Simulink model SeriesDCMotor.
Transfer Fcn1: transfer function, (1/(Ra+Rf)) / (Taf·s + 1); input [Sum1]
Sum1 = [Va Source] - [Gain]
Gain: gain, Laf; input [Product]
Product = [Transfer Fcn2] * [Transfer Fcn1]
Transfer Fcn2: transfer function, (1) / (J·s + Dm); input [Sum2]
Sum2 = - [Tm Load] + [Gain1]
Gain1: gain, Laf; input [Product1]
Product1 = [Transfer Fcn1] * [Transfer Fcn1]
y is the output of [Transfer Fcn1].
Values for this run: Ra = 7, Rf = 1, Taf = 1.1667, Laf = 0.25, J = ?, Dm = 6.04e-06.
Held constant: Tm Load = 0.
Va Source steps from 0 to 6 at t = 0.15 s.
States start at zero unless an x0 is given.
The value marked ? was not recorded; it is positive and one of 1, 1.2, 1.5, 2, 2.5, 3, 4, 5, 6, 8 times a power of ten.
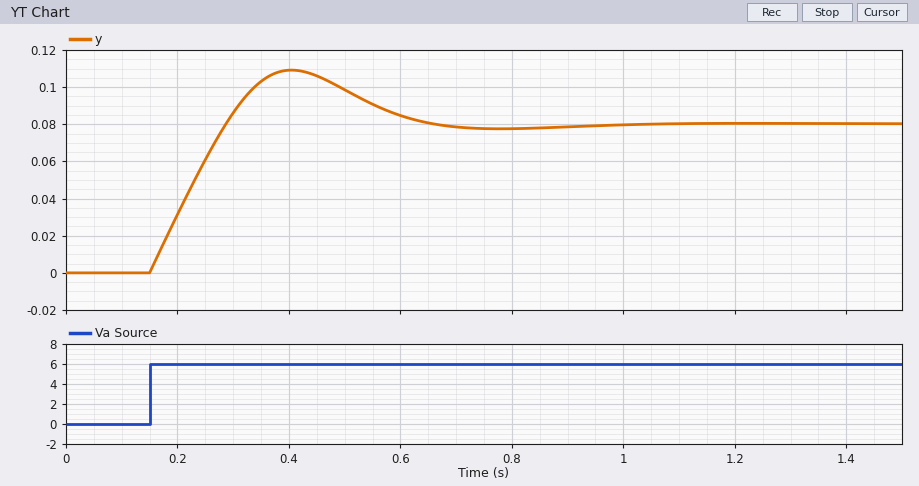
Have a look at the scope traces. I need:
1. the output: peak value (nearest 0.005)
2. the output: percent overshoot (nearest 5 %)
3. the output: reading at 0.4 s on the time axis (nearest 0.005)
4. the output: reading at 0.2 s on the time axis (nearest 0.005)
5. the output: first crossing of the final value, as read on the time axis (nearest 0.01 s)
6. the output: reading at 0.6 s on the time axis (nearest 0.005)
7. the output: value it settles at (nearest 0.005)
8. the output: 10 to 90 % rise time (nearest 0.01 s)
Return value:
0.110
35 %
0.110
0.030
0.29 s
0.085
0.080
0.11 s
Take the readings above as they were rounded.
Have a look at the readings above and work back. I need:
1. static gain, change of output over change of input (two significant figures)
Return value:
0.013
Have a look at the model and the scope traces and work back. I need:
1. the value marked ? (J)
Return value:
1.5e-06
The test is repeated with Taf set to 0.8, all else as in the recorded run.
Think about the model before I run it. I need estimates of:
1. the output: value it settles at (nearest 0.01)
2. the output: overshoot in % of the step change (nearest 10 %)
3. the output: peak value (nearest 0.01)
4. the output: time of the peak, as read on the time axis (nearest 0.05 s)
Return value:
0.08
50 %
0.12
0.35 s
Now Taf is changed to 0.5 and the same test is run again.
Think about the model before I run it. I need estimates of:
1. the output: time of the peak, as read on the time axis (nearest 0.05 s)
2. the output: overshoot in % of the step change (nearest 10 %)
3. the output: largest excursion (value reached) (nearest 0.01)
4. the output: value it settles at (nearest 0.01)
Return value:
0.30 s
60 %
0.13
0.08
